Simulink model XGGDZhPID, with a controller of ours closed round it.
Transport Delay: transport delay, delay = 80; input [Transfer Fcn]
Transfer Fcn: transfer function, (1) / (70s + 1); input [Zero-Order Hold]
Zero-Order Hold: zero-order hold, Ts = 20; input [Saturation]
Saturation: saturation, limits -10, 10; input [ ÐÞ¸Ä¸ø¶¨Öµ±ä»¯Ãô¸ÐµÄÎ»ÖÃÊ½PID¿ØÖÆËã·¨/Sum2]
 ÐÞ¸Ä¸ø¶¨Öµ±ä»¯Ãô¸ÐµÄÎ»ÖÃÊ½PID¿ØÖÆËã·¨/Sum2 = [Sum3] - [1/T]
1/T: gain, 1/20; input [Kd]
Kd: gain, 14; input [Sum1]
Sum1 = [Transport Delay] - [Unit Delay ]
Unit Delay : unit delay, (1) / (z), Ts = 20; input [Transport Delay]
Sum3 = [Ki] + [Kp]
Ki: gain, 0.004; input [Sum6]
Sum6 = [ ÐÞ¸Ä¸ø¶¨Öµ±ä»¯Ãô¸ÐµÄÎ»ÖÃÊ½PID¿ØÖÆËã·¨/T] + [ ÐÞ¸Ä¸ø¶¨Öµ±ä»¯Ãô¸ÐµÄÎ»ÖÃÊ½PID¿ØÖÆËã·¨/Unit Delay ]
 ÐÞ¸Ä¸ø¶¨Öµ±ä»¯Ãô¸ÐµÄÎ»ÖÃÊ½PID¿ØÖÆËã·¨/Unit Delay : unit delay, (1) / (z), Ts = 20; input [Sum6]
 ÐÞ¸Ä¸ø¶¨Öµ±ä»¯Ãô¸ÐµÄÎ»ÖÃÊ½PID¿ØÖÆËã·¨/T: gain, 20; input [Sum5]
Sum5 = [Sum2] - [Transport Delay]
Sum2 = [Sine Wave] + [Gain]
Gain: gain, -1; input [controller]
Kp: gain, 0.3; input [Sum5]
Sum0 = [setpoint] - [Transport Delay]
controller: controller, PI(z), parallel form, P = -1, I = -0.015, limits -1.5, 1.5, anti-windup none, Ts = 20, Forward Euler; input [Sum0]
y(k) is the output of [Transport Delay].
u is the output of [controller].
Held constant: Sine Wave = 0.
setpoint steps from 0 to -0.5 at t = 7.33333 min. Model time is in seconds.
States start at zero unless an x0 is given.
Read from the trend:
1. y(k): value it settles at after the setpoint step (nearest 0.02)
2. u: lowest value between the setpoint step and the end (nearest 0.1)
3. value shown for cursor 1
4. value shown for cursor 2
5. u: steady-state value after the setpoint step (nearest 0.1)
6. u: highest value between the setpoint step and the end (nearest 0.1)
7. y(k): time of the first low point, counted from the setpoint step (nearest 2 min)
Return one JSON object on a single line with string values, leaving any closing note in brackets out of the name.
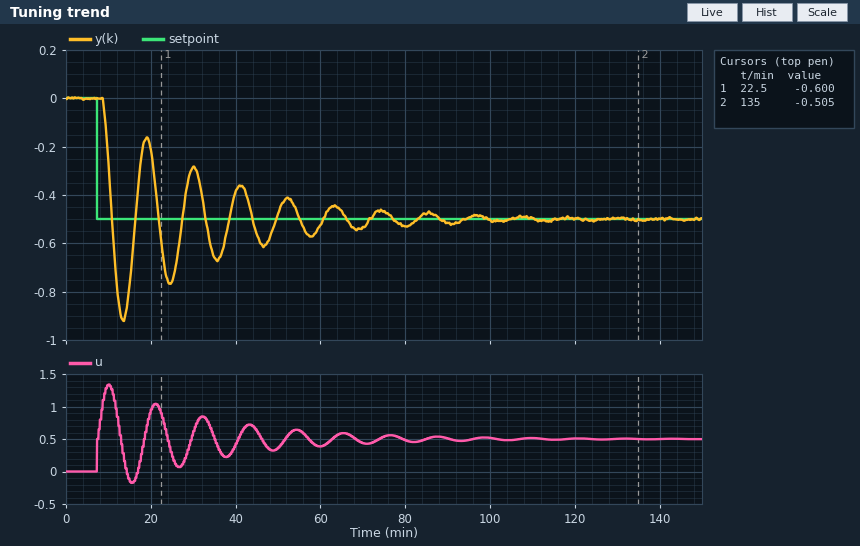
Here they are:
{"y(k): value it settles at after the setpoint step": "-0.50", "u: lowest value between the setpoint step and the end": "-0.2", "value shown for cursor 1": "-0.600", "value shown for cursor 2": "-0.505", "u: steady-state value after the setpoint step": "0.5", "u: highest value between the setpoint step and the end": "1.3", "y(k): time of the first low point, counted from the setpoint step": "6 min"}
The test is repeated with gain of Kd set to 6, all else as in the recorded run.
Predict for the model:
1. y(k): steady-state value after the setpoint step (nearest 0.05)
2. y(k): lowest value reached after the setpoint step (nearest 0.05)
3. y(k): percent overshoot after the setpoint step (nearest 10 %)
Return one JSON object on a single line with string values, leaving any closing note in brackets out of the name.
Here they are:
{"y(k): steady-state value after the setpoint step": "-0.50", "y(k): lowest value reached after the setpoint step": "-0.95", "y(k): percent overshoot after the setpoint step": "90 %"}
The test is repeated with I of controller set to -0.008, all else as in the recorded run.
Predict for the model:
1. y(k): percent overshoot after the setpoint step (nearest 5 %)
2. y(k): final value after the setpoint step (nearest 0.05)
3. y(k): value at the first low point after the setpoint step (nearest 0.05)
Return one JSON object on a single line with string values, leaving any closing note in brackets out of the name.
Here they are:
{"y(k): percent overshoot after the setpoint step": "30 %", "y(k): final value after the setpoint step": "-0.50", "y(k): value at the first low point after the setpoint step": "-0.65"}
